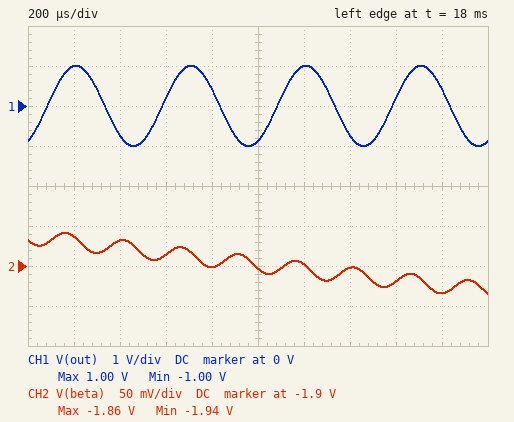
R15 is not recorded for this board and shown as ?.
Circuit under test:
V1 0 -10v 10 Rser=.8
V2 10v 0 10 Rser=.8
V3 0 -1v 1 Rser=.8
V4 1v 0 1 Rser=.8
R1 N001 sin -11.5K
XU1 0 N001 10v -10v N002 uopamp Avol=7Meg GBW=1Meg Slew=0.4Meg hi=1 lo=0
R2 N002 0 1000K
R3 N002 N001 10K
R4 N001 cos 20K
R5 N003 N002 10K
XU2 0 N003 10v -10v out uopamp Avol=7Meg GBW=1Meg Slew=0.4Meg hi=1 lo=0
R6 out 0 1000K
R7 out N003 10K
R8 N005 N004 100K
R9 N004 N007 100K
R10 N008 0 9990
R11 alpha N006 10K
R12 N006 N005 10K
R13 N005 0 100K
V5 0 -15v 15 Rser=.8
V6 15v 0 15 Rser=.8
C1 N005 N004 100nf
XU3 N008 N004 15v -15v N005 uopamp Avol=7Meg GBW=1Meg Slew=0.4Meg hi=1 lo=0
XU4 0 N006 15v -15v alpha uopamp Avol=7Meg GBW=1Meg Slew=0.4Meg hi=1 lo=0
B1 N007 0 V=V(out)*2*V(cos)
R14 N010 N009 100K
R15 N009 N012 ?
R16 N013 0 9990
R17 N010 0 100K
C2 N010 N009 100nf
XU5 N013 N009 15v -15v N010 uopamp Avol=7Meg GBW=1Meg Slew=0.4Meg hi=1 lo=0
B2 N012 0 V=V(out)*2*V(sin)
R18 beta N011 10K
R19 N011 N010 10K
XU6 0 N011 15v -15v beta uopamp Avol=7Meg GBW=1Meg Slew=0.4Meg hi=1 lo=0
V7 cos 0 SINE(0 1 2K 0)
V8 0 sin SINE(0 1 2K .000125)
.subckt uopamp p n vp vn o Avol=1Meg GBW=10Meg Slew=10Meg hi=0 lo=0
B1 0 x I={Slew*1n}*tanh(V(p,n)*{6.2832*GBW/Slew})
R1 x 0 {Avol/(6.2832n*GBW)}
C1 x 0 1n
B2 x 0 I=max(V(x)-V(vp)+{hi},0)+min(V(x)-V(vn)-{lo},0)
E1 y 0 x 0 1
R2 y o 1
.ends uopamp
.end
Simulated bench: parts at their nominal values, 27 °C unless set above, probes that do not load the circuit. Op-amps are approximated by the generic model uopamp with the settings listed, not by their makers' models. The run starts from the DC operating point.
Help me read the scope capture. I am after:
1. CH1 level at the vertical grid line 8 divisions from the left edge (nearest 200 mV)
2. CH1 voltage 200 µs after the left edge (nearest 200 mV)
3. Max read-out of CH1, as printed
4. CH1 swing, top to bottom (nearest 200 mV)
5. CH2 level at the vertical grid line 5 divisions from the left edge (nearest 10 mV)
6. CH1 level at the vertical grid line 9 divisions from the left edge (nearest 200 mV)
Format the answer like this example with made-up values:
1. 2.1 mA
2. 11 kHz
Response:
1. 200 mV
2. 1.0 V
3. 1.00 V
4. 2.0 V
5. -1.90 V
6. 400 mV
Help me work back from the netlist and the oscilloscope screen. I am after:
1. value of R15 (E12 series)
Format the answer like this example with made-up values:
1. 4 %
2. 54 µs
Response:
1. 39 kΩ
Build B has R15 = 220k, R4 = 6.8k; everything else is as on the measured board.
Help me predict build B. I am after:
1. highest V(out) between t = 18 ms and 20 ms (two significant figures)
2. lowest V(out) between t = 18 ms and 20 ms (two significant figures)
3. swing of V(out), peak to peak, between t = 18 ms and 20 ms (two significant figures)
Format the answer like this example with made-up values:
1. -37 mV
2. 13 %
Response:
1. 1.7 V
2. -1.7 V
3. 3.4 V
